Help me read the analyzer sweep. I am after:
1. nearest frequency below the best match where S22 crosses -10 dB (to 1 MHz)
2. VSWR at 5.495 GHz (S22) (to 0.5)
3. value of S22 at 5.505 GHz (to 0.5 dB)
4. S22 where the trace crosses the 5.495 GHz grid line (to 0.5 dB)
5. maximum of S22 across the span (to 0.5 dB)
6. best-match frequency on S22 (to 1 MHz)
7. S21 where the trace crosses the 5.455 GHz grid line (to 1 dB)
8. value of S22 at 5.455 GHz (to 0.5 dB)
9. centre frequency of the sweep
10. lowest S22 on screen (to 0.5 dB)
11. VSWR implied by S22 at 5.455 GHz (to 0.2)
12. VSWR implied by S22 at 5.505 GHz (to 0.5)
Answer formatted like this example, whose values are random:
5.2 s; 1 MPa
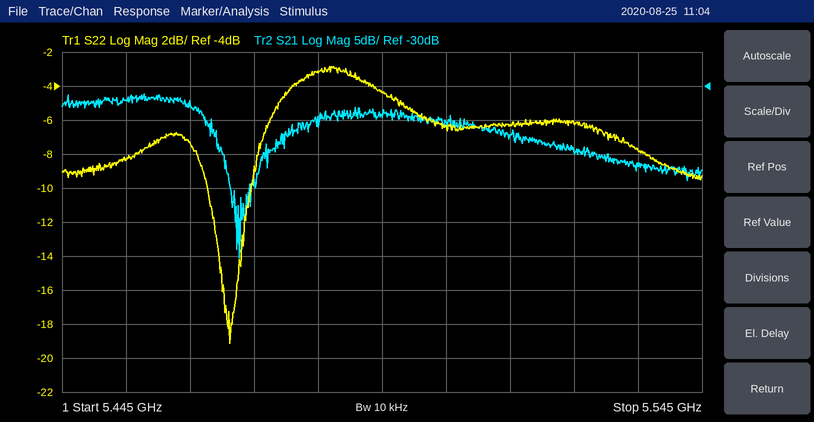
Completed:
5.468 GHz; 4.0; -6.5 dB; -4.5 dB; -3.0 dB; 5.471 GHz; -32 dB; -8.5 dB; 5.495 GHz; -19.0 dB; 2.2; 3.0
